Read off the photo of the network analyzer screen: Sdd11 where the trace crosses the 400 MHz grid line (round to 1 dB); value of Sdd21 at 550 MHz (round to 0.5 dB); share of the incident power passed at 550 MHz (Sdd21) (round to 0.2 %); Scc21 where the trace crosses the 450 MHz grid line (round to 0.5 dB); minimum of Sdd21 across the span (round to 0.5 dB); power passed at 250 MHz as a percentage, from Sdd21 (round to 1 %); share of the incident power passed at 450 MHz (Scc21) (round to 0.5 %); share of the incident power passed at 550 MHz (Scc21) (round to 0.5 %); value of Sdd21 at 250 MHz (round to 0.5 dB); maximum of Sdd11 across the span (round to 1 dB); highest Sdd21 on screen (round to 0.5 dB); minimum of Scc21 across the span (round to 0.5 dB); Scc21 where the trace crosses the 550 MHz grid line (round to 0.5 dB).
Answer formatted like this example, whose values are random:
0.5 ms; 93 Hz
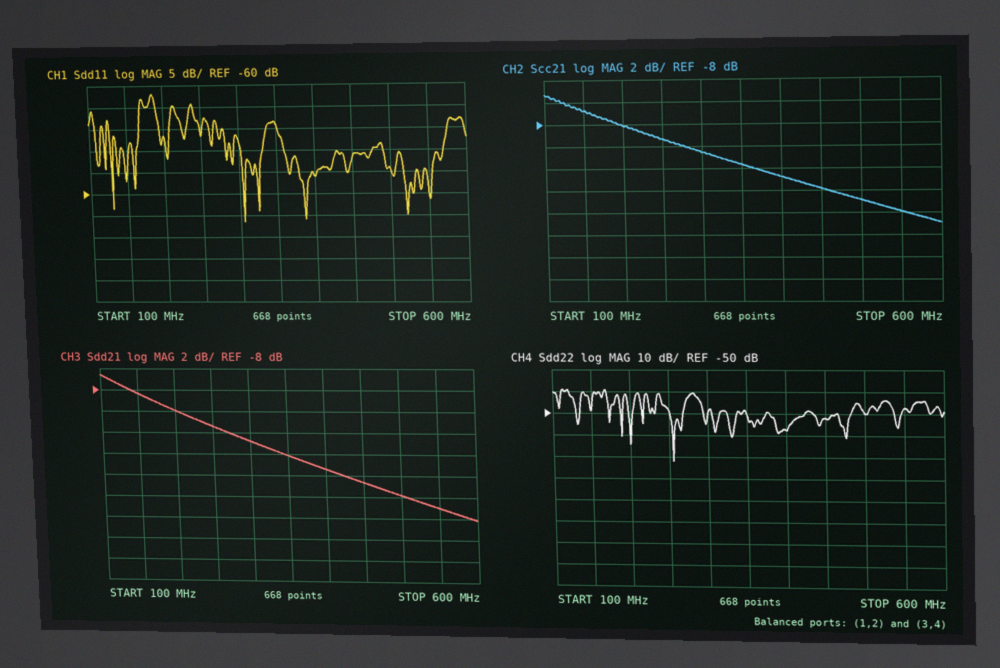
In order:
-56 dB; -19.0 dB; 1.2 %; -14.0 dB; -20.0 dB; 7 %; 4.0 %; 2.5 %; -11.5 dB; -37 dB; -6.5 dB; -17.0 dB; -16.0 dB
